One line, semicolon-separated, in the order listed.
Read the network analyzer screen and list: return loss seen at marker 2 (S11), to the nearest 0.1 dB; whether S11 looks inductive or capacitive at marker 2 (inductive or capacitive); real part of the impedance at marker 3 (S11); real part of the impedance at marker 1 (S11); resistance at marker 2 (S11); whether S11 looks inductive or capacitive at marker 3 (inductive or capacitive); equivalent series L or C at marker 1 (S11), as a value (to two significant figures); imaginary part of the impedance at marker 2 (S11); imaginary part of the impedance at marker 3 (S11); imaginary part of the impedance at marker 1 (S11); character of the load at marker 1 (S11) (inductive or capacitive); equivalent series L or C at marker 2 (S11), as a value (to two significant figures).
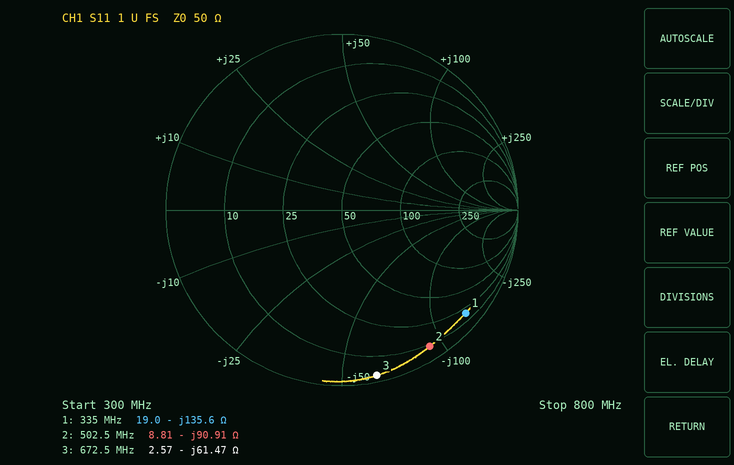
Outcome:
0.7 dB; capacitive; 2.57 Ω; 19.0 Ω; 8.81 Ω; capacitive; 3.5 pF; -90.91 Ω; -61.47 Ω; -135.6 Ω; capacitive; 3.5 pF
